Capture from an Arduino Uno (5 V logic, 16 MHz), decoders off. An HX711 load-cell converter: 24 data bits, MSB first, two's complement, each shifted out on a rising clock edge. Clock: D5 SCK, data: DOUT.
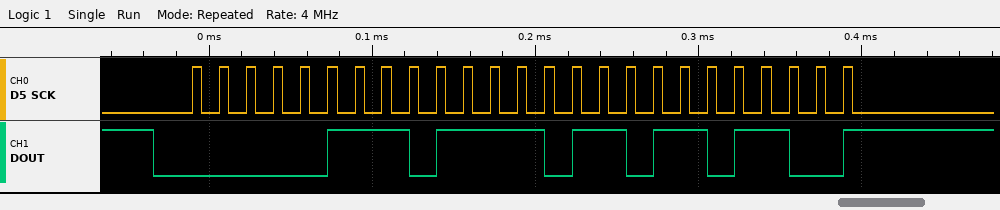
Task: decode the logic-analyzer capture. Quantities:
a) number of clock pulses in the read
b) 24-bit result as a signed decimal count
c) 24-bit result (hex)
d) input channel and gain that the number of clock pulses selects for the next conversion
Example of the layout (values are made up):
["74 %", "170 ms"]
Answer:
["25", "490348", "0x077B6C", "channel A, gain 128"]
